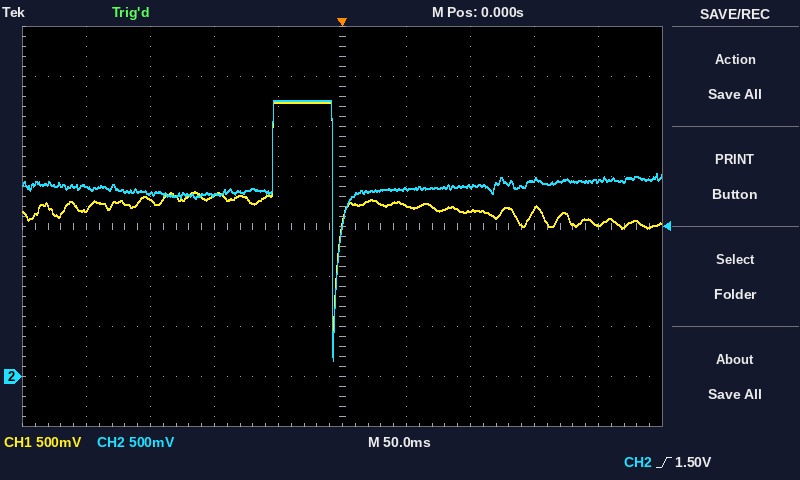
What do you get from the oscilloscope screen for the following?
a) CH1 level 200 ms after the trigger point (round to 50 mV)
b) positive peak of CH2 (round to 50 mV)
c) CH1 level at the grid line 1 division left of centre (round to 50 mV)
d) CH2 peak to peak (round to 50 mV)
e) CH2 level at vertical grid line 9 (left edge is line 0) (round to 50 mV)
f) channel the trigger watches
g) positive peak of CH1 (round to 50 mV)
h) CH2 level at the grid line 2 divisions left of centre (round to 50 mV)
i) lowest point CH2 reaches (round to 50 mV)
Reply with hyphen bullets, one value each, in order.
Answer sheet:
- 1.50 V
- 2.75 V
- 2.75 V
- 2.60 V
- 1.95 V
- CH2
- 2.75 V
- 1.80 V
- 150 mV
